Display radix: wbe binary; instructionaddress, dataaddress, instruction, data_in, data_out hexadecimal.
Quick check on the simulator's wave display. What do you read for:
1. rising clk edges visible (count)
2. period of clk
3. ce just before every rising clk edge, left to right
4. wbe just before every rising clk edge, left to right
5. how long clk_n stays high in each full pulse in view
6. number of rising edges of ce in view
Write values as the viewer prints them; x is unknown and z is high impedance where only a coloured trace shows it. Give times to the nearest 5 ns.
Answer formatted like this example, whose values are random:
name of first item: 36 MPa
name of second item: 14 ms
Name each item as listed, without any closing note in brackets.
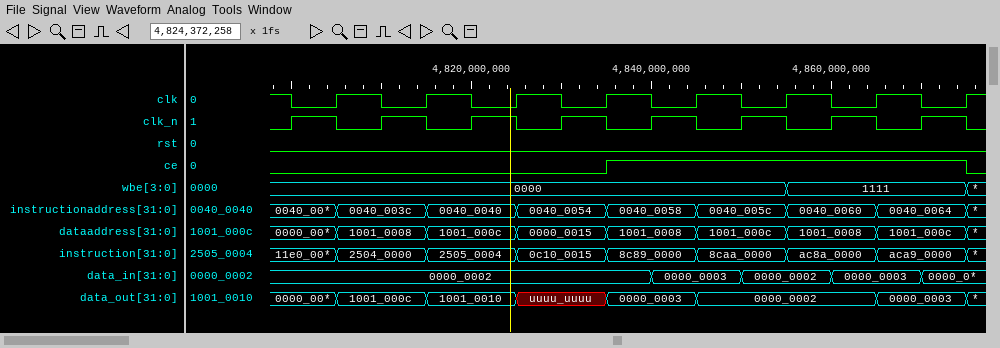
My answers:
rising clk edges visible: 8
period of clk: 10 ns
ce just before every rising clk edge, left to right: 0 0 0 0 1 1 1 1
wbe just before every rising clk edge, left to right: 0000, 0000, 0000, 0000, 0000, 0000, 1111, 1111
how long clk_n stays high in each full pulse in view: 5 ns, 5 ns, 5 ns, 5 ns, 5 ns, 5 ns, 5 ns, 5 ns
number of rising edges of ce in view: 1
